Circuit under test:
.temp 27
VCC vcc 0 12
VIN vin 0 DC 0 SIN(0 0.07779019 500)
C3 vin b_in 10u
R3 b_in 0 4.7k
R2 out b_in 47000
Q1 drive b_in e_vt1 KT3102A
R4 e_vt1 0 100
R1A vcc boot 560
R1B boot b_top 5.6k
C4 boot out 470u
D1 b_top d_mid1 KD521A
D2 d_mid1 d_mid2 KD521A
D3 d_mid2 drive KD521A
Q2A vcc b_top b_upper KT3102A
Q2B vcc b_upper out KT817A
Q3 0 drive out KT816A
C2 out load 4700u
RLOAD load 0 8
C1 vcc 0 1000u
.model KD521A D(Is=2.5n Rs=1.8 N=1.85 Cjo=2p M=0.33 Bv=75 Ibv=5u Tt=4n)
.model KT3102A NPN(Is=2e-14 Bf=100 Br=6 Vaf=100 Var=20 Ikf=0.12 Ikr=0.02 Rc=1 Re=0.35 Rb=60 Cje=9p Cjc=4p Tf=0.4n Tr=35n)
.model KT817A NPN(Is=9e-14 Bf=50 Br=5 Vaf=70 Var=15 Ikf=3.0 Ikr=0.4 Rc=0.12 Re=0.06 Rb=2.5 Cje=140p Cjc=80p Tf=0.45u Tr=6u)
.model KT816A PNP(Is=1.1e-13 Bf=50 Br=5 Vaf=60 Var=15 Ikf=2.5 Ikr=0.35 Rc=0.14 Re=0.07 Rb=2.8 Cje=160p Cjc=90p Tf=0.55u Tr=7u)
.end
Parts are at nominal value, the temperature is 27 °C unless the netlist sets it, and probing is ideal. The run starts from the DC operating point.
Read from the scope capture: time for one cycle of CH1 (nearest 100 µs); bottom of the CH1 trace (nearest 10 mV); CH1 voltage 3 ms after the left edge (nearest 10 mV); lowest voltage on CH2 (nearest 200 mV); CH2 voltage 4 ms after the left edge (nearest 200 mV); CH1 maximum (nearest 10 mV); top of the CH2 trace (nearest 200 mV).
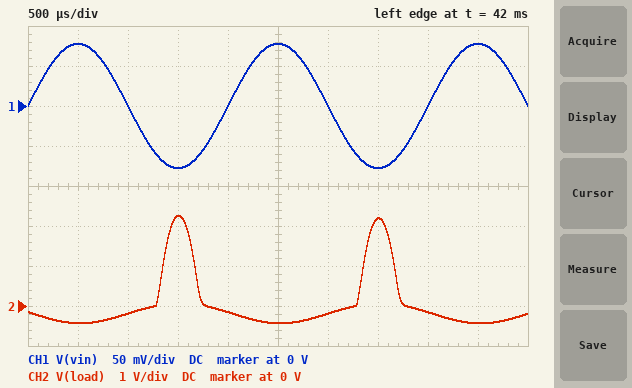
2.0 ms
-80 mV
0 V
-400 mV
-200 mV
80 mV
2.2 V
